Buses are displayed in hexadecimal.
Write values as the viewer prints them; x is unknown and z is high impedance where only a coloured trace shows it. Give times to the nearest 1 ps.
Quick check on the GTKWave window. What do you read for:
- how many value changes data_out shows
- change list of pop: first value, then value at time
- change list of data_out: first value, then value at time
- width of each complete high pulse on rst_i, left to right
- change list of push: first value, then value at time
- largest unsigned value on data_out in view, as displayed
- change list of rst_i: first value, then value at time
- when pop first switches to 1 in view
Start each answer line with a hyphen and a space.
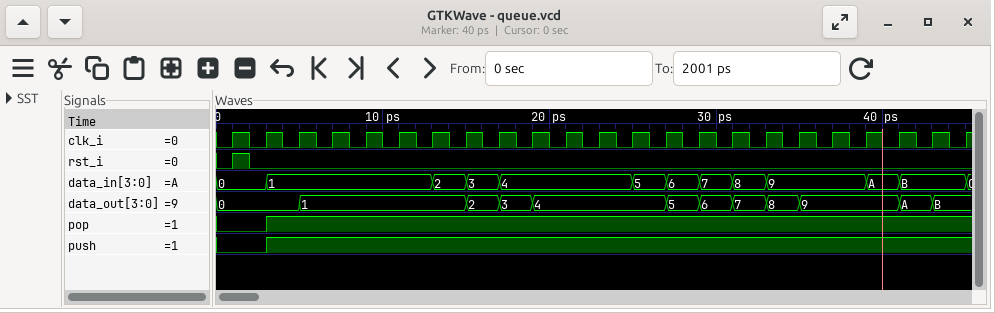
- 11
- 0, 1 at 3 ps
- 0, 1 at 5 ps, 2 at 15 ps, 3 at 17 ps, 4 at 19 ps, 5 at 27 ps, 6 at 29 ps, 7 at 31 ps, 8 at 33 ps, 9 at 35 ps, A at 41 ps, B at 43 ps
- 1 ps
- 0, 1 at 3 ps
- B
- 0, 1 at 1 ps, 0 at 2 ps
- 3 ps
